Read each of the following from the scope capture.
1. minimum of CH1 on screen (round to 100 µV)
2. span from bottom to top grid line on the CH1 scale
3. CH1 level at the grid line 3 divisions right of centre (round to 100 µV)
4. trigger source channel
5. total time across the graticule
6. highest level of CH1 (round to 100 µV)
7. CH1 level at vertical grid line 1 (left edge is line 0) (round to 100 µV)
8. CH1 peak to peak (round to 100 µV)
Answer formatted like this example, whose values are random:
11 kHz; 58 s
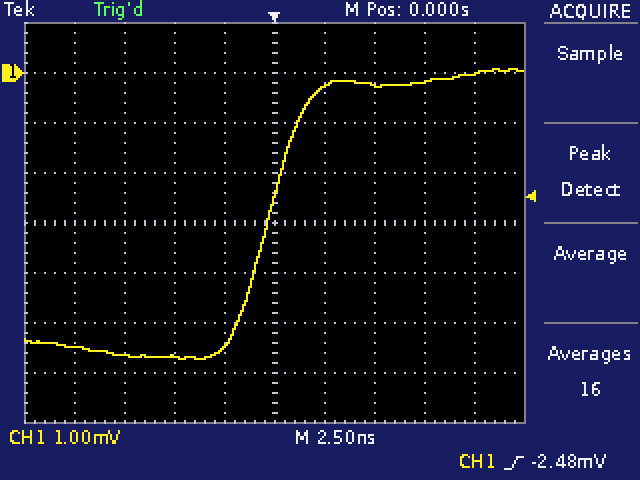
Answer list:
-5.7 mV; 8 mV; -200 µV; CH1; 25 ns; 100 µV; -5.5 mV; 5.8 mV
